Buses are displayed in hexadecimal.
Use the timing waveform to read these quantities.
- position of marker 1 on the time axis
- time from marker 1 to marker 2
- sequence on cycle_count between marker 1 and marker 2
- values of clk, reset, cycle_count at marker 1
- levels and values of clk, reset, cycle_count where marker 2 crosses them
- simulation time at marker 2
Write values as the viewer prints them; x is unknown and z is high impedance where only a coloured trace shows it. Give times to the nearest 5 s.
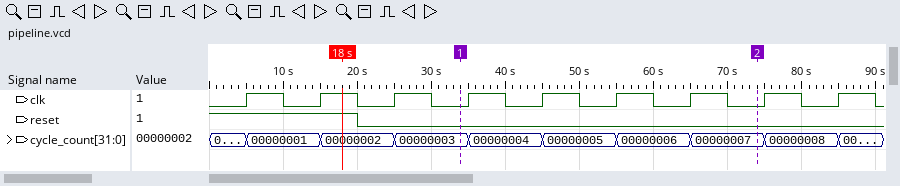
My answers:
35 s
40 s
00000003, 00000004, 00000005, 00000006, 00000007
clk=0, reset=0, cycle_count=00000003
clk=0, reset=0, cycle_count=00000007
75 s
